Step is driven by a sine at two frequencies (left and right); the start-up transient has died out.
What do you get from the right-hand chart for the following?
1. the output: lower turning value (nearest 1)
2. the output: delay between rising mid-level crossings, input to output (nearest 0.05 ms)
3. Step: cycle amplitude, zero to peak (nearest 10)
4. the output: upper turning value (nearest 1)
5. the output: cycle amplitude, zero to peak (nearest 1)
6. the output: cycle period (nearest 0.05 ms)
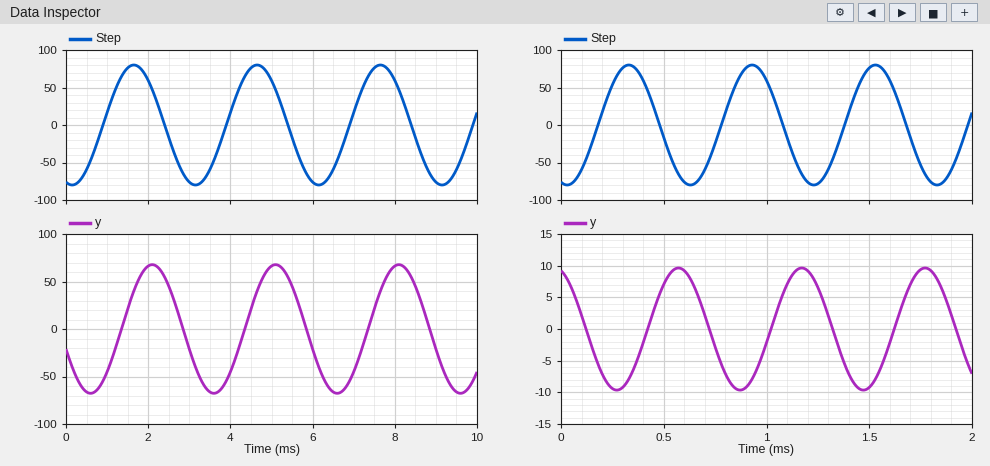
-10
0.25 ms
80
10
10
0.60 ms
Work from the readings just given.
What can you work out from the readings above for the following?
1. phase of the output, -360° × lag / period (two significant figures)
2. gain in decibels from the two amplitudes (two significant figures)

-150°
-18 dB
